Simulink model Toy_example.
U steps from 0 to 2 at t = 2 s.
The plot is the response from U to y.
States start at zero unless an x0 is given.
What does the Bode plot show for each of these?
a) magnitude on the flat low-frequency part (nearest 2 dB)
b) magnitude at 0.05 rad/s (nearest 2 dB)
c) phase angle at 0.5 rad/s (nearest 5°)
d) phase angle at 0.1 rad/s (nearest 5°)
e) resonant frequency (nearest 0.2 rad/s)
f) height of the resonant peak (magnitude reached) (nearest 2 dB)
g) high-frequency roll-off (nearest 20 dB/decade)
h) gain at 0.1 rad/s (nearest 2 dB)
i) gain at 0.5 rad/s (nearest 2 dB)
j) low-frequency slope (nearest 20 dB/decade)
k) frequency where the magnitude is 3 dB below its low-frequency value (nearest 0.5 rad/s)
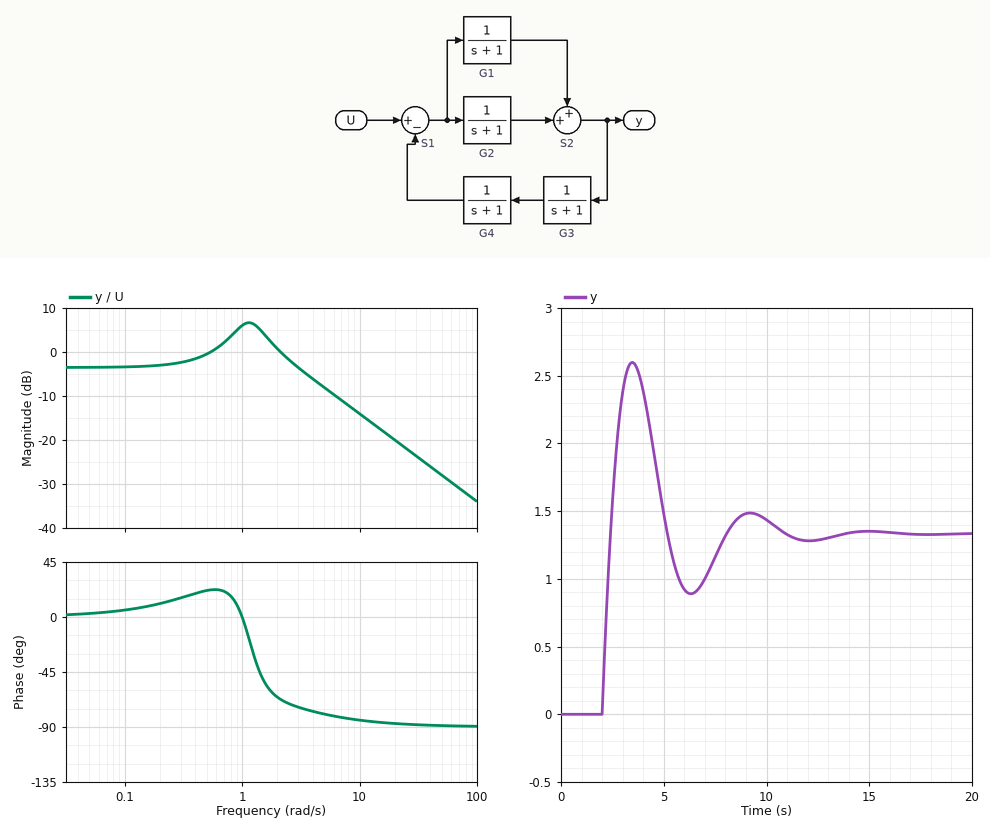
-4 dB
-4 dB
20°
5°
1.2 rad/s
6 dB
-20 dB/decade
-4 dB
0 dB
0 dB/decade
4.0 rad/s
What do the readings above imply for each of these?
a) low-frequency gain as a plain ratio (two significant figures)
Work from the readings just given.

0.63
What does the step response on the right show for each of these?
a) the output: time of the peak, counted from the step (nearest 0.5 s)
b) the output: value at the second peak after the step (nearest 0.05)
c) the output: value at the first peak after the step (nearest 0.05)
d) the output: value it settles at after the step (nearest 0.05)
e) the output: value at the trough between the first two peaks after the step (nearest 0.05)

1.5 s
1.50
2.60
1.35
0.90
